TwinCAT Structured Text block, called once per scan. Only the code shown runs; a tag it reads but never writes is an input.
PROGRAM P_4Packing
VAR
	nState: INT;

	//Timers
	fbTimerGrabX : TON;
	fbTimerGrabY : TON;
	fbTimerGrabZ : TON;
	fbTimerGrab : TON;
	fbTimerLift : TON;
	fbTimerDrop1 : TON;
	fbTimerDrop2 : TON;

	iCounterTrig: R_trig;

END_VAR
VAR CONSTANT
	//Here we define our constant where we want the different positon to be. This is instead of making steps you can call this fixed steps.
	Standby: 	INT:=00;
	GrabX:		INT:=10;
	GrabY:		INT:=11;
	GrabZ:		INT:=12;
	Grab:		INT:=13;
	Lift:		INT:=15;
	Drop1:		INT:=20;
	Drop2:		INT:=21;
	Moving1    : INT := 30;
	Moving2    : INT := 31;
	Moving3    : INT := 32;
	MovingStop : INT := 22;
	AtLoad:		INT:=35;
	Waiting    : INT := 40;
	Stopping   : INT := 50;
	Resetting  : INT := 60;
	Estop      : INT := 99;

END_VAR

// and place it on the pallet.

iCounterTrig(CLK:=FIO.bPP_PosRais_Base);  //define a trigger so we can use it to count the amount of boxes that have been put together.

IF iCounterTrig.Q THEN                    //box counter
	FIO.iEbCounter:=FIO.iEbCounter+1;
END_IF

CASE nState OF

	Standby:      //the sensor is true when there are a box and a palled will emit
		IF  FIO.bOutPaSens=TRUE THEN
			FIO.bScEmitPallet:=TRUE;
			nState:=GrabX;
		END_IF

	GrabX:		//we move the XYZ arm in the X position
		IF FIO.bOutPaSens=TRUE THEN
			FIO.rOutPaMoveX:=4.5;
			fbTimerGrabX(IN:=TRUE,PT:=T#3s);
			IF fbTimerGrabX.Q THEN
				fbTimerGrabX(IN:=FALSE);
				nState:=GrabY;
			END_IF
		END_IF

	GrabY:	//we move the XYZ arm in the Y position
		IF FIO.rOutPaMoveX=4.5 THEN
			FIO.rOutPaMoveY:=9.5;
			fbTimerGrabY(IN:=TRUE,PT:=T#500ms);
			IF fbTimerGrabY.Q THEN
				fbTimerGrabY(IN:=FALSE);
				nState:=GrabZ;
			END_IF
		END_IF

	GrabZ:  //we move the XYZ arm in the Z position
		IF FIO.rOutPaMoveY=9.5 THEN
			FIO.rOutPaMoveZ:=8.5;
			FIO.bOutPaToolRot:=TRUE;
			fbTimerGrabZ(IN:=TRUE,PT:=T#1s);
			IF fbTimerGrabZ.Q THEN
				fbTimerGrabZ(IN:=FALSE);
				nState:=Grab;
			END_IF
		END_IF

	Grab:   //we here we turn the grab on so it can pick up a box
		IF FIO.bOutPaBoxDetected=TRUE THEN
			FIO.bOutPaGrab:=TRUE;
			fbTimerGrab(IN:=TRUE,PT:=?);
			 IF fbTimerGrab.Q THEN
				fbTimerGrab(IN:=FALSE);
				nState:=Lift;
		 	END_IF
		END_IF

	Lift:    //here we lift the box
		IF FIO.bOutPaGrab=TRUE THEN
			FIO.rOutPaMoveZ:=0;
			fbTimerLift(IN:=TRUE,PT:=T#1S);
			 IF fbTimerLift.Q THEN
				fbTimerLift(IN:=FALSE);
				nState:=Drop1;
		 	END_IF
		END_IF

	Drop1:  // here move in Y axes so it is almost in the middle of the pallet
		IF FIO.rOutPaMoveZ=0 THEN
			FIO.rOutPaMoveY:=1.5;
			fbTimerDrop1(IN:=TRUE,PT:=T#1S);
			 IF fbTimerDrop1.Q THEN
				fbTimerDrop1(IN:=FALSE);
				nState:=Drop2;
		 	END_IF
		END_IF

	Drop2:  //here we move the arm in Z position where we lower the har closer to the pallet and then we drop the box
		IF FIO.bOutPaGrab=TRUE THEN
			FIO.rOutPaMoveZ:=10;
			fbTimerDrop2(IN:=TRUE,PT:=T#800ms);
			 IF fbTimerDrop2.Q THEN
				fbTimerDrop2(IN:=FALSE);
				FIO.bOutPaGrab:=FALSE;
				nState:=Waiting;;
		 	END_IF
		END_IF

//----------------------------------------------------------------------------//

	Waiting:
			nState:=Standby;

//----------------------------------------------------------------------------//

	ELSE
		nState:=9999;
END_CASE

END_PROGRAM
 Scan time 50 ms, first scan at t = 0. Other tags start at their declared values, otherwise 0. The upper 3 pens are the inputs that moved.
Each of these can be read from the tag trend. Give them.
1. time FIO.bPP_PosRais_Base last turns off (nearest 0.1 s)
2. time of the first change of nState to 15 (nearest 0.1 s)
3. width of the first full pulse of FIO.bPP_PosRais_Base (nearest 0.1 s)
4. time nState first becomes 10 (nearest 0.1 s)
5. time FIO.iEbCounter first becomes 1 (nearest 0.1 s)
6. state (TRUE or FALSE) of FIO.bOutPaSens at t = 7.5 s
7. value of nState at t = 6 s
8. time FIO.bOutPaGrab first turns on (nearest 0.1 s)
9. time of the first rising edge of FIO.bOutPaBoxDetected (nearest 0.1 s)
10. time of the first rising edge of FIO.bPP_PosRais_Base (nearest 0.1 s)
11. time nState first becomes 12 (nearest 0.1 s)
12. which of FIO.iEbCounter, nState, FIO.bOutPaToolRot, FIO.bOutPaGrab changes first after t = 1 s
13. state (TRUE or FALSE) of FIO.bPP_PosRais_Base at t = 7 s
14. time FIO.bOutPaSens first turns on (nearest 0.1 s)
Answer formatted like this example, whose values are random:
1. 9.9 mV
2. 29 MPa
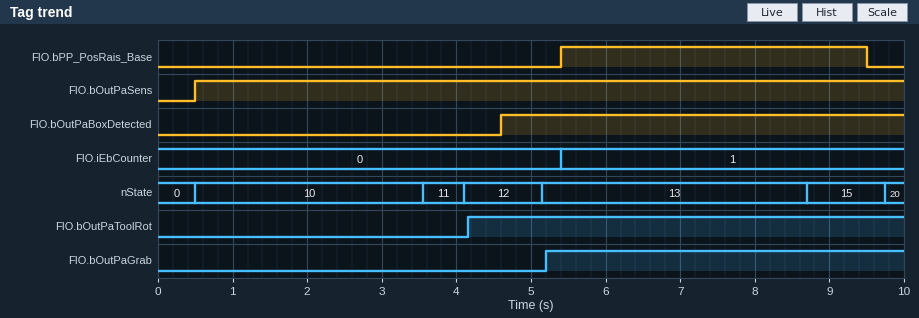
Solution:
1. 9.5 s
2. 8.7 s
3. 4.1 s
4. 0.5 s
5. 5.4 s
6. TRUE
7. 13
8. 5.2 s
9. 4.6 s
10. 5.4 s
11. 4.1 s
12. nState
13. TRUE
14. 0.5 s
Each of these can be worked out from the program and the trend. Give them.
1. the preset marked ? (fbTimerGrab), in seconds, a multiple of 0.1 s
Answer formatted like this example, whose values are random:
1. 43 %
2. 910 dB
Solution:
1. 3.5 s
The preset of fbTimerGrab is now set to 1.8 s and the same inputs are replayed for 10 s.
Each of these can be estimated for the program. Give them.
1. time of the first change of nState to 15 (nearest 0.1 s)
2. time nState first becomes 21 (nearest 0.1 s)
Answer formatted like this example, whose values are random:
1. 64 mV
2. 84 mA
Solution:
1. 7.0 s
2. 9.1 s
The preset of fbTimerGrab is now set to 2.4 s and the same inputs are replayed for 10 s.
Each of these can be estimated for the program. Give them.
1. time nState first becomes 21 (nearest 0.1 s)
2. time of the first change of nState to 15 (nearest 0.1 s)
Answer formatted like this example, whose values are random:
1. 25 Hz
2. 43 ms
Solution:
1. 9.7 s
2. 7.6 s
